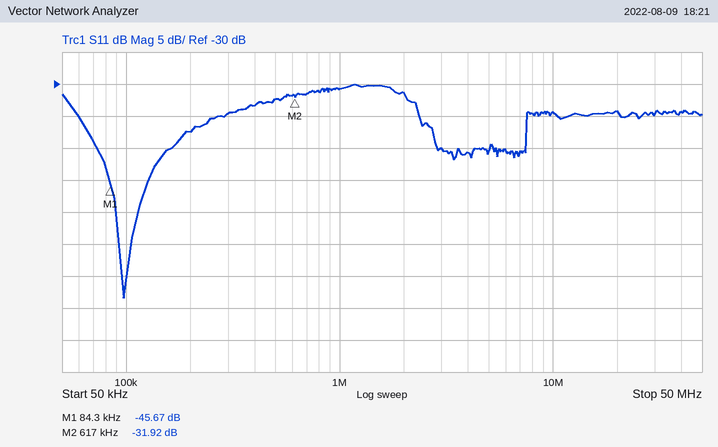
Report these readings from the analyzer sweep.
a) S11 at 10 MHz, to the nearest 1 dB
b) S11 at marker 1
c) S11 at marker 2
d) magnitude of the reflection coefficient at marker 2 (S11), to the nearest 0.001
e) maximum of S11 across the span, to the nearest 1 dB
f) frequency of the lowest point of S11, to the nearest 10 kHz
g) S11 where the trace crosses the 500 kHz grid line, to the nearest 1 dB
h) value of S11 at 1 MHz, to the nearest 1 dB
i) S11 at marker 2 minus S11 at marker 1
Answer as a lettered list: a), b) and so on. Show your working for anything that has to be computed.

a) -34 dB
b) -45.67 dB
c) -31.92 dB
d) 10^(-31.92/20) ≈ 0.025
e) -30 dB
f) 100 kHz
g) -32 dB
h) -31 dB
i) -31.92 − (-45.67) = 13.75 dB
